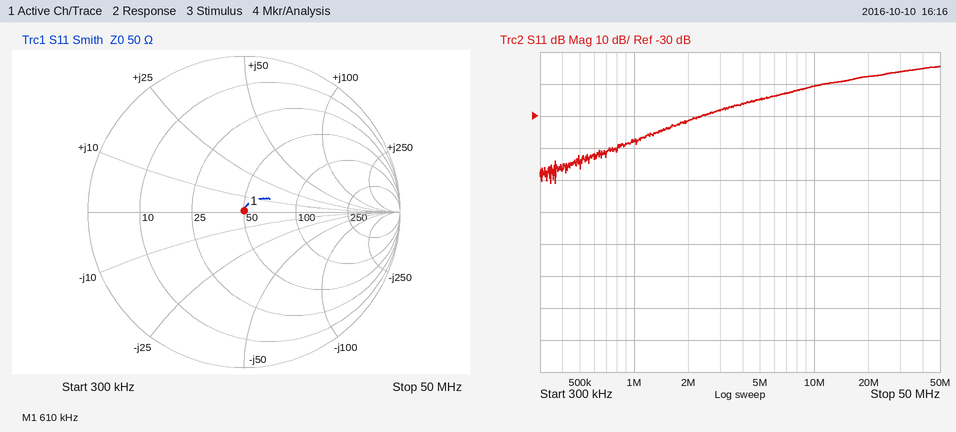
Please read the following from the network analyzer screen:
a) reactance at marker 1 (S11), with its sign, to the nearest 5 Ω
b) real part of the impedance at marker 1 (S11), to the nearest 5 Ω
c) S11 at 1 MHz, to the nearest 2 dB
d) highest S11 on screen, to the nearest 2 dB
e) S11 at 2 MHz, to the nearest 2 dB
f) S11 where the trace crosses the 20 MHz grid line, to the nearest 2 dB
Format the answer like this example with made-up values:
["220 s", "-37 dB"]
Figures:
["0 Ω", "50 Ω", "-38 dB", "-14 dB", "-32 dB", "-18 dB"]
